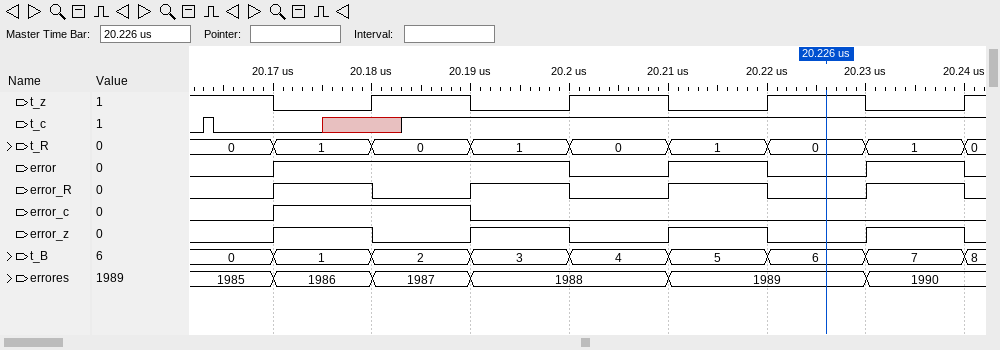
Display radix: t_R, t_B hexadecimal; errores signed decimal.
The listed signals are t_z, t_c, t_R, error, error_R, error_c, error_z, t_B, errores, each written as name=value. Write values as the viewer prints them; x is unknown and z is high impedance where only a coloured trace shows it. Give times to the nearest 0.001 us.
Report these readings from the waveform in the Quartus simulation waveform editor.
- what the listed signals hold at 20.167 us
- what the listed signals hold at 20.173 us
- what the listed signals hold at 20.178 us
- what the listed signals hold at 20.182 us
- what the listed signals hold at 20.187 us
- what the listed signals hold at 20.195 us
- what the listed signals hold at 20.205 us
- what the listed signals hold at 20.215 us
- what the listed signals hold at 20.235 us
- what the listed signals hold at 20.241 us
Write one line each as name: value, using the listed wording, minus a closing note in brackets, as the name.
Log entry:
what the listed signals hold at 20.167 us: t_z=1, t_c=0, t_R=0, error=0, error_R=0, error_c=0, error_z=0, t_B=0, errores=1985
what the listed signals hold at 20.173 us: t_z=0, t_c=0, t_R=1, error=1, error_R=1, error_c=1, error_z=1, t_B=1, errores=1986
what the listed signals hold at 20.178 us: t_z=0, t_c=x, t_R=1, error=1, error_R=1, error_c=1, error_z=1, t_B=1, errores=1986
what the listed signals hold at 20.182 us: t_z=1, t_c=x, t_R=0, error=1, error_R=0, error_c=1, error_z=0, t_B=2, errores=1987
what the listed signals hold at 20.187 us: t_z=1, t_c=1, t_R=0, error=1, error_R=0, error_c=1, error_z=0, t_B=2, errores=1987
what the listed signals hold at 20.195 us: t_z=0, t_c=1, t_R=1, error=1, error_R=1, error_c=0, error_z=1, t_B=3, errores=1988
what the listed signals hold at 20.205 us: t_z=1, t_c=1, t_R=0, error=0, error_R=0, error_c=0, error_z=0, t_B=4, errores=1988
what the listed signals hold at 20.215 us: t_z=0, t_c=1, t_R=1, error=1, error_R=1, error_c=0, error_z=1, t_B=5, errores=1989
what the listed signals hold at 20.235 us: t_z=0, t_c=1, t_R=1, error=1, error_R=1, error_c=0, error_z=1, t_B=7, errores=1990
what the listed signals hold at 20.241 us: t_z=1, t_c=1, t_R=0, error=0, error_R=0, error_c=0, error_z=0, t_B=8, errores=1990
